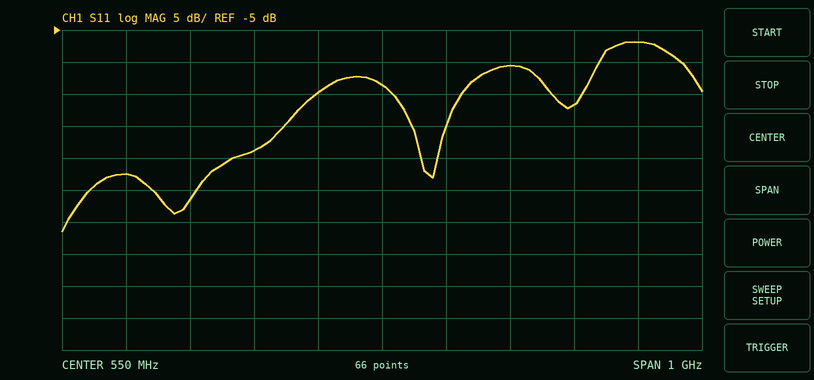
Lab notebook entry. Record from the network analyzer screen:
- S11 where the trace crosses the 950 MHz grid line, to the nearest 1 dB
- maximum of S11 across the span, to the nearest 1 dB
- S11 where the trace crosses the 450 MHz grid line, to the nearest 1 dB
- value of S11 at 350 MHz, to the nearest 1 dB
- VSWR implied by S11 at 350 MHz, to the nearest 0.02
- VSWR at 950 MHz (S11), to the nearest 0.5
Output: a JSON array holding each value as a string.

["-7 dB", "-7 dB", "-15 dB", "-24 dB", "1.14", "2.5"]
